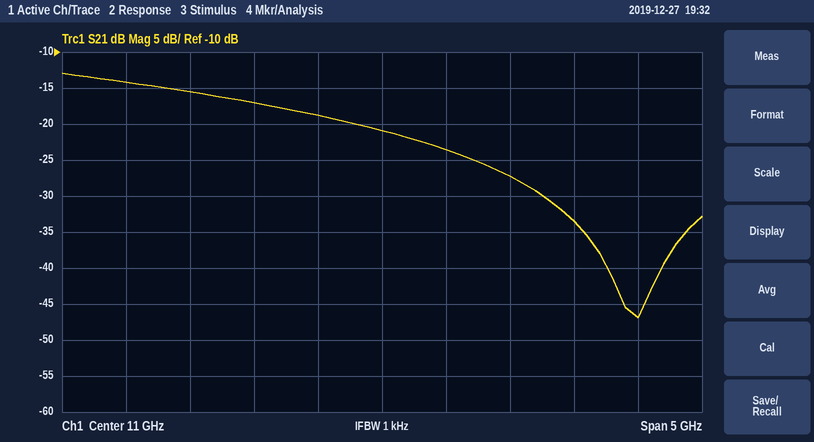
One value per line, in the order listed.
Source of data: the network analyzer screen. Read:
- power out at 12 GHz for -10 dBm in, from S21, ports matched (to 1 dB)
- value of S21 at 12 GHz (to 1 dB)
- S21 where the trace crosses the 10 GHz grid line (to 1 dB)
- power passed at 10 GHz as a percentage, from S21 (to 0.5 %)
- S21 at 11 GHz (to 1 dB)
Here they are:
-37 dBm
-27 dB
-17 dB
2.0 %
-21 dB
